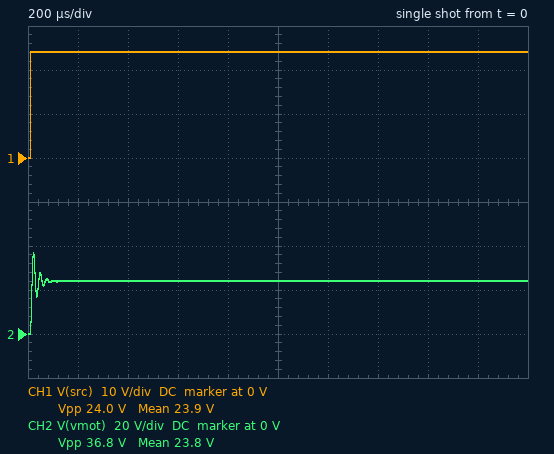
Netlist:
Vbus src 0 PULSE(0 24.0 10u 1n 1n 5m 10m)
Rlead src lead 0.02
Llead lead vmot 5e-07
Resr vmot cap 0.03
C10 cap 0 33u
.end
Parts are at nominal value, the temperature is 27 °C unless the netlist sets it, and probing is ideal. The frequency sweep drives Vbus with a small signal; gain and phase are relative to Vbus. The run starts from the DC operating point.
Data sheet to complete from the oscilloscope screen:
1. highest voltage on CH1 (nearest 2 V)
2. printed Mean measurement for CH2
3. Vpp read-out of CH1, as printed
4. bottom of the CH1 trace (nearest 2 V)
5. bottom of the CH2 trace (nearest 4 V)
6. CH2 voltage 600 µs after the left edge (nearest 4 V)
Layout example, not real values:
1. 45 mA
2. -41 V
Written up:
1. 24 V
2. 23.8 V
3. 24.0 V
4. 0 V
5. 0 V
6. 24 V
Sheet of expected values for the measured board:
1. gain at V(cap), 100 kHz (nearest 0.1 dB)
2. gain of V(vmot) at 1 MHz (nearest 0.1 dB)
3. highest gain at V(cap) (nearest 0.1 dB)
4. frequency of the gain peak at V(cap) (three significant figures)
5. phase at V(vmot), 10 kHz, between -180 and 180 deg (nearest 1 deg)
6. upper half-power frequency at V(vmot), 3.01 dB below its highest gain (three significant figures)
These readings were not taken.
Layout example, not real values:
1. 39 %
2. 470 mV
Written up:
1. -15.0 dB
2. -40.3 dB
3. 8.0 dB
4. 37.5 kHz
5. -3 deg
6. 45.1 kHz
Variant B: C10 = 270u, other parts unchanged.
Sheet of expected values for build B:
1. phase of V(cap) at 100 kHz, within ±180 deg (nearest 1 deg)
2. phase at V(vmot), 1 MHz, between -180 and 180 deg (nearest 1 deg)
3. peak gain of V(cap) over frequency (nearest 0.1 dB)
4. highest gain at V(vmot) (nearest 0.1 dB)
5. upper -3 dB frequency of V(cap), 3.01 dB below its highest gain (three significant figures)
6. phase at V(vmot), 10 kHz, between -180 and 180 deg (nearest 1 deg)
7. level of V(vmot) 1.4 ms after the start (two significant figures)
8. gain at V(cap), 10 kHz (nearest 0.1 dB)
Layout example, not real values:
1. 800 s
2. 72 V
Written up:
1. -171 deg
2. -90 deg
3. 0.5 dB
4. 1.3 dB
5. 15.4 kHz
6. -34 deg
7. 24 V
8. 0.3 dB
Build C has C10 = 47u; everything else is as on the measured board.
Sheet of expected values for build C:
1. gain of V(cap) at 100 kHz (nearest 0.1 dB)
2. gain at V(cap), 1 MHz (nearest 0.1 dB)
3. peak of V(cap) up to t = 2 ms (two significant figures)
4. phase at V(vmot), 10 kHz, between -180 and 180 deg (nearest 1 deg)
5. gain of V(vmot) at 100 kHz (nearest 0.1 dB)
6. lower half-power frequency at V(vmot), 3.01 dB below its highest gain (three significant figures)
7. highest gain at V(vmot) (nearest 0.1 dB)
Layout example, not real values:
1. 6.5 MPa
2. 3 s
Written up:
1. -18.5 dB
2. -59.3 dB
3. 35 V
4. -4 deg
5. -16.0 dB
6. 21.5 kHz
7. 6.9 dB
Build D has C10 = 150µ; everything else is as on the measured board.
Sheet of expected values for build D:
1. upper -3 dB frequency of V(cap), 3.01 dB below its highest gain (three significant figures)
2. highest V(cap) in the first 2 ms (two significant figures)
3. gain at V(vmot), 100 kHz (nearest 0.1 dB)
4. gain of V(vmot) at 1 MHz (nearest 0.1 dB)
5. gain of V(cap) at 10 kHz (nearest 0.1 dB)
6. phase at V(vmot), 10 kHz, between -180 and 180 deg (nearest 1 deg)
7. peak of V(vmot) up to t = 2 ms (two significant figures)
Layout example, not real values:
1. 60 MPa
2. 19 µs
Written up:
1. 21.8 kHz
2. 29 V
3. -19.7 dB
4. -40.4 dB
5. 1.4 dB
6. -18 deg
7. 30 V
